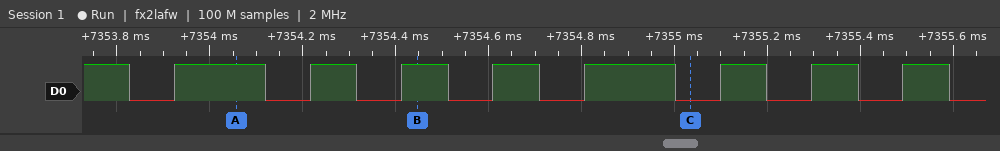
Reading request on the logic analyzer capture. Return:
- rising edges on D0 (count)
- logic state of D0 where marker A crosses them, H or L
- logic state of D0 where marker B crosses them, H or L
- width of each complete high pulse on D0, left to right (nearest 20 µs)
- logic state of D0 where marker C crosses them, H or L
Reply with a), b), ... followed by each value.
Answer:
a) 8
b) D0=H
c) D0=H
d) 200 µs, 100 µs, 100 µs, 100 µs, 200 µs, 100 µs, 100 µs, 100 µs
e) D0=L
